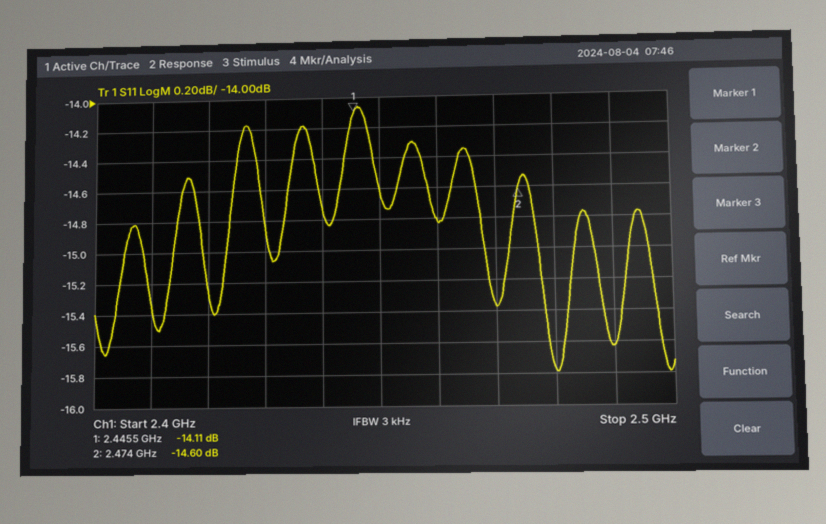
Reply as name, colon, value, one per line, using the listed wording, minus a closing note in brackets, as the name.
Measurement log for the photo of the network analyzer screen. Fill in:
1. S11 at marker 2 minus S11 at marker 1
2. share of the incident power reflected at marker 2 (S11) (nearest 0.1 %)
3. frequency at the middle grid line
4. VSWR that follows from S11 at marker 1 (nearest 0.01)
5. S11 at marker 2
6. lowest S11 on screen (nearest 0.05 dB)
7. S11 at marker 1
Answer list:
S11 at marker 2 minus S11 at marker 1: -0.49 dB
share of the incident power reflected at marker 2 (S11): 3.5 %
frequency at the middle grid line: 2.45 GHz
VSWR that follows from S11 at marker 1: 1.49
S11 at marker 2: -14.60 dB
lowest S11 on screen: -15.80 dB
S11 at marker 1: -14.11 dB
